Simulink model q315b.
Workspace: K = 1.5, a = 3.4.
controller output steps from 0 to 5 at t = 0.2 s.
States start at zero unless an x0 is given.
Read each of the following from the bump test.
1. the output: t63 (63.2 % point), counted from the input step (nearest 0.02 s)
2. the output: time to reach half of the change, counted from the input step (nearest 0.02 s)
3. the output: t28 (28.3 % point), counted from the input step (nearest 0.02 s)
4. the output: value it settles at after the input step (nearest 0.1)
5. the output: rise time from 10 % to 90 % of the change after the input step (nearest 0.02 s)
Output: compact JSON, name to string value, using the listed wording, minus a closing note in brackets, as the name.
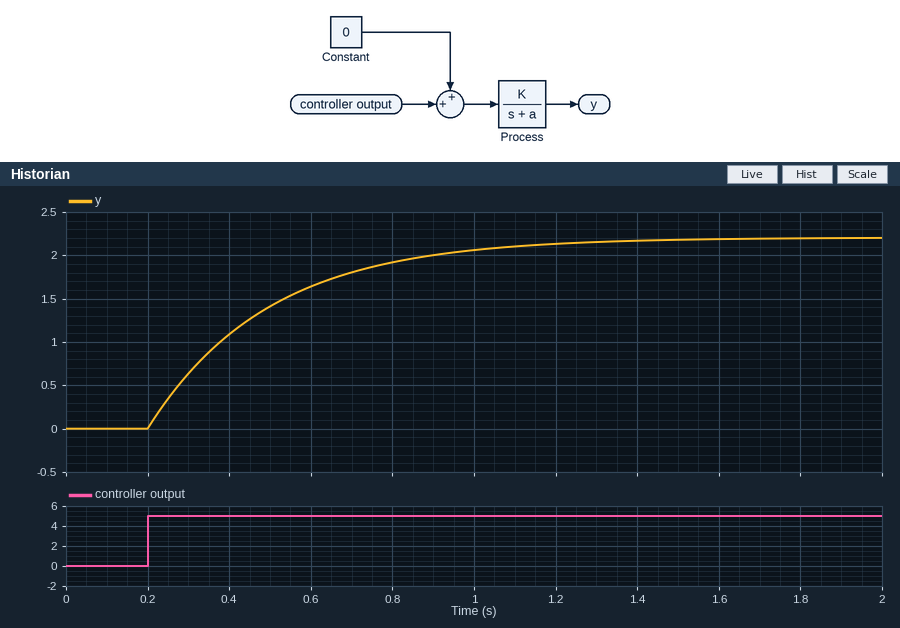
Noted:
{"the output: t63 (63.2 % point), counted from the input step": "0.30 s", "the output: time to reach half of the change, counted from the input step": "0.20 s", "the output: t28 (28.3 % point), counted from the input step": "0.10 s", "the output: value it settles at after the input step": "2.2", "the output: rise time from 10 % to 90 % of the change after the input step": "0.64 s"}
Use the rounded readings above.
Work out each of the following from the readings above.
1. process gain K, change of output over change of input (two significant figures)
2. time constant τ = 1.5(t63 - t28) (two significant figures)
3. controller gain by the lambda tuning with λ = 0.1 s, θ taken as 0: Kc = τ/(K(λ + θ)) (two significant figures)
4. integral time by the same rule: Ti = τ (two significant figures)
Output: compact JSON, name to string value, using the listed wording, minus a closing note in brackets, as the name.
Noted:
{"process gain K, change of output over change of input": "0.44", "time constant τ = 1.5(t63 - t28)": "0.30 s", "controller gain by the lambda tuning with λ = 0.1 s, θ taken as 0: Kc = τ/(K(λ + θ))": "6.8", "integral time by the same rule: Ti = τ": "0.30 s"}
